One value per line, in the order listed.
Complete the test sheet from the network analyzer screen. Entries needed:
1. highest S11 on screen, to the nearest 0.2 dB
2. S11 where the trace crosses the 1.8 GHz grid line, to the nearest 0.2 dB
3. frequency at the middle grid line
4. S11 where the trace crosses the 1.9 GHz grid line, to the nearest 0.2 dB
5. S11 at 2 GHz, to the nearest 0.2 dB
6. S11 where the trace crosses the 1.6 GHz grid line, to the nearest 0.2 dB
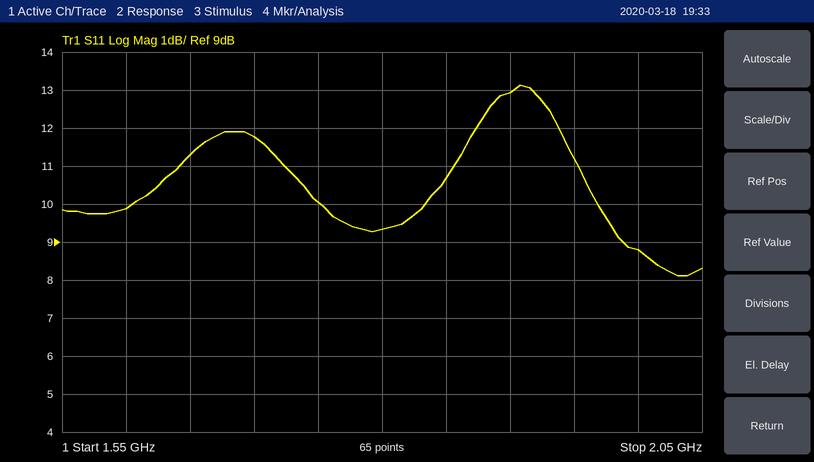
13.2 dB
9.4 dB
1.8 GHz
13.0 dB
8.8 dB
9.8 dB
